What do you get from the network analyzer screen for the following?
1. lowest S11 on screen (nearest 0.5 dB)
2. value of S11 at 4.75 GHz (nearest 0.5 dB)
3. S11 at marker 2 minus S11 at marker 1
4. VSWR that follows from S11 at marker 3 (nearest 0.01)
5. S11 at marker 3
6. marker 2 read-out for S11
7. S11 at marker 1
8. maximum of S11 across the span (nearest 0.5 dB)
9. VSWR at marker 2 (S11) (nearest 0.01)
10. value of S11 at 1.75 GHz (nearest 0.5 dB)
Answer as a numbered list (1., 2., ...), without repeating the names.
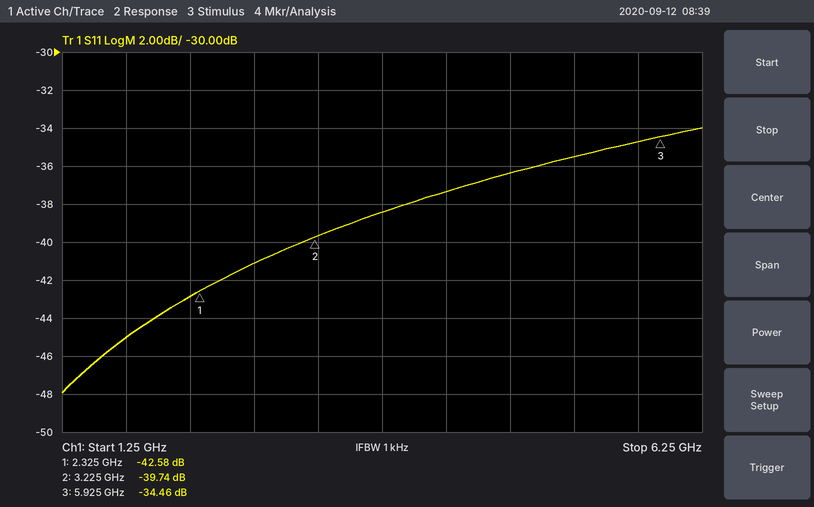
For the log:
1. -48.0 dB
2. -36.5 dB
3. 2.84 dB
4. 1.04
5. -34.46 dB
6. -39.74 dB
7. -42.58 dB
8. -34.0 dB
9. 1.02
10. -45.0 dB
